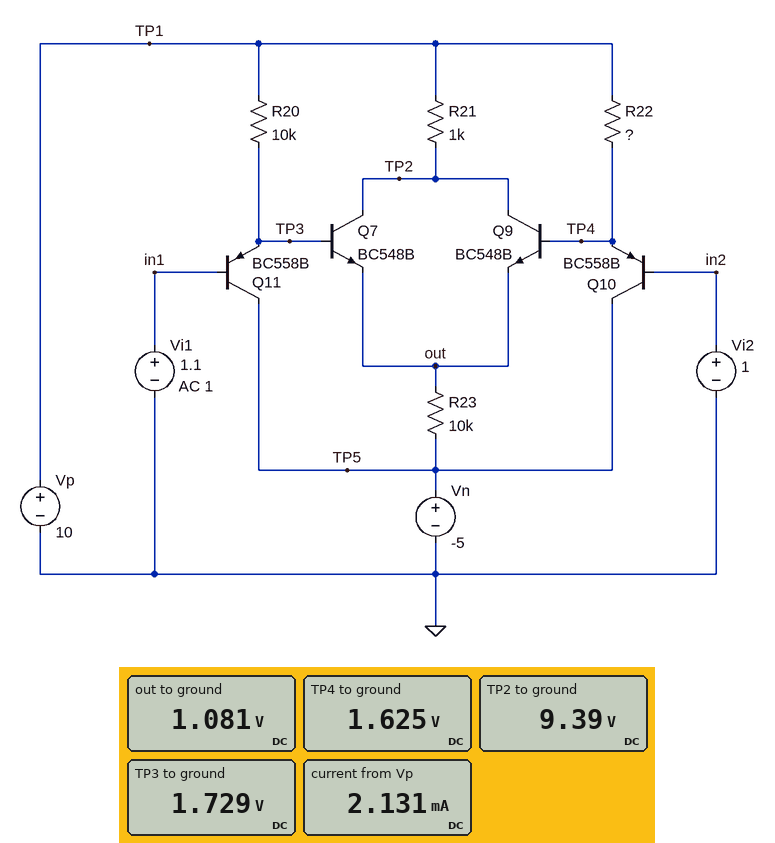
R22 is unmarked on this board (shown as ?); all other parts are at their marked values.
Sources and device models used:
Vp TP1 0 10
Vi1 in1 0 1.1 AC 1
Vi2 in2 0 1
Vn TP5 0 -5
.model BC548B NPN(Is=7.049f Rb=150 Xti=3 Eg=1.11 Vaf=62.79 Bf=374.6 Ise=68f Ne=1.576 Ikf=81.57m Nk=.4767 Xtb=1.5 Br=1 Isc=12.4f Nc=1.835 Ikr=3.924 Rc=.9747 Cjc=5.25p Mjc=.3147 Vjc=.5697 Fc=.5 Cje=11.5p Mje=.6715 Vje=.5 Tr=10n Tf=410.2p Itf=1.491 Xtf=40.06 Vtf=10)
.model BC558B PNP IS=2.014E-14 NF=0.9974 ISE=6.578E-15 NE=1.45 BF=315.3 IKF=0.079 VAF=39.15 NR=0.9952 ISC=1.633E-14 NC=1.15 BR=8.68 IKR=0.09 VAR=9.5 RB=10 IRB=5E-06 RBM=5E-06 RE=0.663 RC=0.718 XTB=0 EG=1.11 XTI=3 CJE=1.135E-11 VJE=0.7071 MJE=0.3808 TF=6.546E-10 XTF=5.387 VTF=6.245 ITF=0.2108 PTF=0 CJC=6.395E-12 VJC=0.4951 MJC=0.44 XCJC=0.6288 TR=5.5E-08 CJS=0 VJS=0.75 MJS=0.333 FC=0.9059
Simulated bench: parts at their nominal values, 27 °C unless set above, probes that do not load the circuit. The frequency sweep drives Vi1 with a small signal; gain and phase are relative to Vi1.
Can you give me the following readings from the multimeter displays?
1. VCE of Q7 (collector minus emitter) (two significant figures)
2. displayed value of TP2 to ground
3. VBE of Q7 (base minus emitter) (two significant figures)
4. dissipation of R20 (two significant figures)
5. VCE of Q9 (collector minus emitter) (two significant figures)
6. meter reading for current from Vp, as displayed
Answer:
8.3 V
9.39 V
650 mV
6.8 mW
8.3 V
2.131 mA
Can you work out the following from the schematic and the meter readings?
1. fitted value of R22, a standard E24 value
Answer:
12 kΩ
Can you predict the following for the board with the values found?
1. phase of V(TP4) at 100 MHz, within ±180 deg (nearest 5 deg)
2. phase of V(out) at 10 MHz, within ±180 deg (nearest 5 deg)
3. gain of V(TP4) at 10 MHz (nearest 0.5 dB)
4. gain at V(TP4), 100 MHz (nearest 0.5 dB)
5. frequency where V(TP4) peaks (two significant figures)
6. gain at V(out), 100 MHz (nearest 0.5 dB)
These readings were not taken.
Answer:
-20 deg
-10 deg
-23.5 dB
-24.0 dB
23 MHz
-7.5 dB
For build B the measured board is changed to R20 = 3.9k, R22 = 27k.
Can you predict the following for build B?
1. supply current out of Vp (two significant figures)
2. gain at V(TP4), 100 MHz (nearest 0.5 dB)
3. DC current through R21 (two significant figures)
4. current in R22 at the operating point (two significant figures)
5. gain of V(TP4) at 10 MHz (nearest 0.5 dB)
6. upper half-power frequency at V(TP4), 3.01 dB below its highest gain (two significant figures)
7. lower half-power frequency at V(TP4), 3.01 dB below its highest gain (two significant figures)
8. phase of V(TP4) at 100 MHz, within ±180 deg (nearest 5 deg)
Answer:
3.0 mA
-19.5 dB
610 µA
310 µA
-18.0 dB
69 MHz
9.3 MHz
-35 deg
